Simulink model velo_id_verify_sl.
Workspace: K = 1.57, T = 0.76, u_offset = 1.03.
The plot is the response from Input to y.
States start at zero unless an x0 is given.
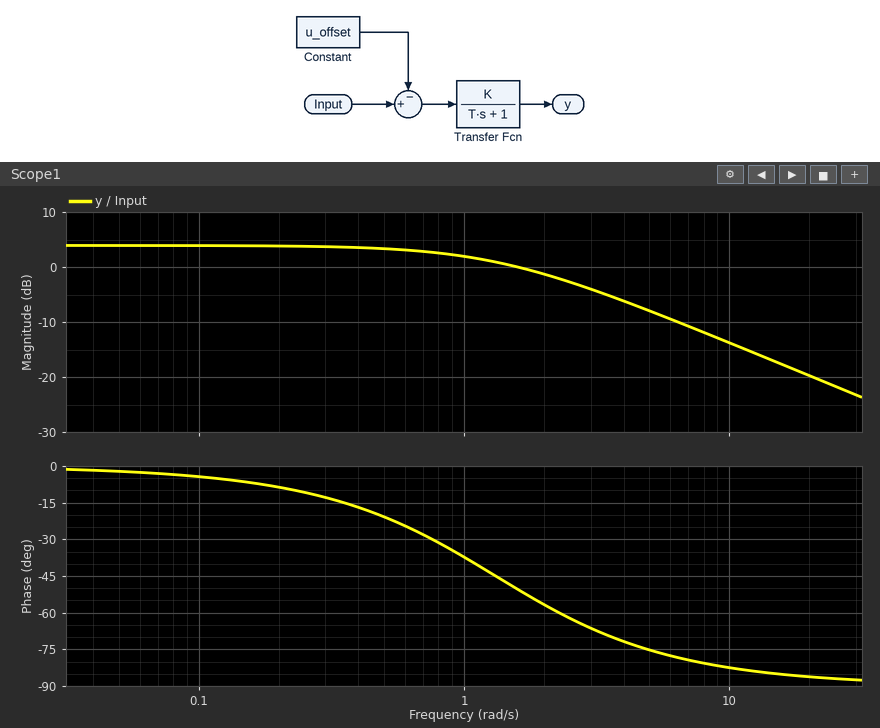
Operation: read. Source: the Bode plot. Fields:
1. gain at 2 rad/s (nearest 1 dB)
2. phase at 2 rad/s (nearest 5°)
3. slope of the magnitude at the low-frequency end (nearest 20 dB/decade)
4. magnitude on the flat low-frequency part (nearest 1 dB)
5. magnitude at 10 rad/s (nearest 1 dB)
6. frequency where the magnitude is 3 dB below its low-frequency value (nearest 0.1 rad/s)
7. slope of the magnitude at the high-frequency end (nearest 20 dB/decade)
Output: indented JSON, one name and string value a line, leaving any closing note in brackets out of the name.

{
  "gain at 2 rad/s": "-1 dB",
  "phase at 2 rad/s": "-55°",
  "slope of the magnitude at the low-frequency end": "0 dB/decade",
  "magnitude on the flat low-frequency part": "4 dB",
  "magnitude at 10 rad/s": "-14 dB",
  "frequency where the magnitude is 3 dB below its low-frequency value": "1.3 rad/s",
  "slope of the magnitude at the high-frequency end": "-20 dB/decade"
}
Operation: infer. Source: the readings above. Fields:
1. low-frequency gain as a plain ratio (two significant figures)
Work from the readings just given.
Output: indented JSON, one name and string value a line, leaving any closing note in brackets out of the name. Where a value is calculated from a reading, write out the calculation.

{
  "low-frequency gain as a plain ratio": "10^(4 / 20) = 1.6"
}
